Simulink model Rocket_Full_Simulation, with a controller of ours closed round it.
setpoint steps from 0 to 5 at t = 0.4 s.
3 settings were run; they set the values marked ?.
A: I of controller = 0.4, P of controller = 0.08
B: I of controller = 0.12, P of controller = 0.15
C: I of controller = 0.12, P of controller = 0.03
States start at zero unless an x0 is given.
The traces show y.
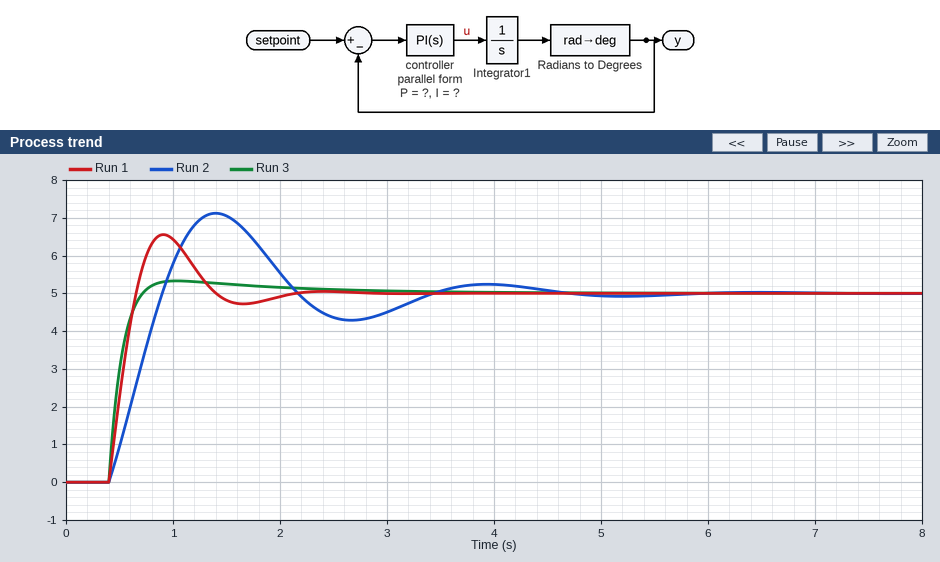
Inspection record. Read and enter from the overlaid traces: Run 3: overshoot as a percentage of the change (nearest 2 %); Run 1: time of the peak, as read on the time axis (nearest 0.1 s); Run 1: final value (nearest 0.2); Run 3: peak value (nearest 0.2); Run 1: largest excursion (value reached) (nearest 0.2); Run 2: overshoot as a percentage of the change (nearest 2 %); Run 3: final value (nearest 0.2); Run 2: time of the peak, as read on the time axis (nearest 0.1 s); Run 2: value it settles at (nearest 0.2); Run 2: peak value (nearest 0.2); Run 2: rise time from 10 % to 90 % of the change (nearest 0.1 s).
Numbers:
6 %
0.9 s
5.0
5.4
6.6
42 %
5.0
1.4 s
5.0
7.2
0.4 s
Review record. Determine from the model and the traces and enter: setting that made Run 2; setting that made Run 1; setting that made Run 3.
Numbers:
C
A
B
